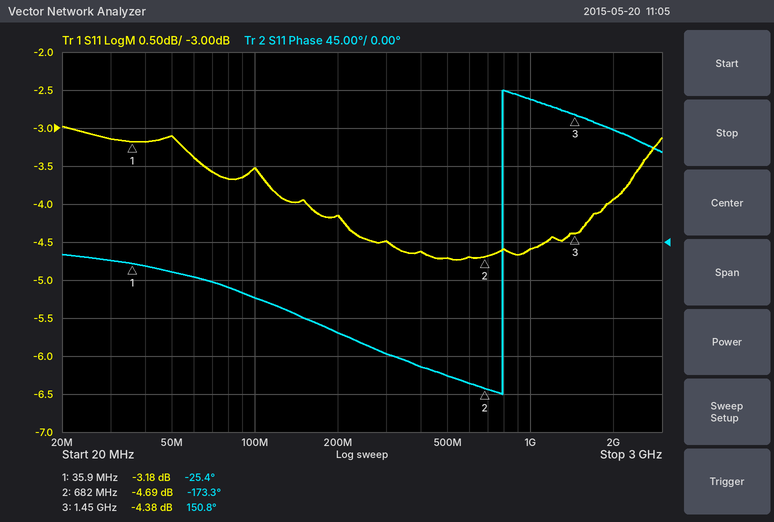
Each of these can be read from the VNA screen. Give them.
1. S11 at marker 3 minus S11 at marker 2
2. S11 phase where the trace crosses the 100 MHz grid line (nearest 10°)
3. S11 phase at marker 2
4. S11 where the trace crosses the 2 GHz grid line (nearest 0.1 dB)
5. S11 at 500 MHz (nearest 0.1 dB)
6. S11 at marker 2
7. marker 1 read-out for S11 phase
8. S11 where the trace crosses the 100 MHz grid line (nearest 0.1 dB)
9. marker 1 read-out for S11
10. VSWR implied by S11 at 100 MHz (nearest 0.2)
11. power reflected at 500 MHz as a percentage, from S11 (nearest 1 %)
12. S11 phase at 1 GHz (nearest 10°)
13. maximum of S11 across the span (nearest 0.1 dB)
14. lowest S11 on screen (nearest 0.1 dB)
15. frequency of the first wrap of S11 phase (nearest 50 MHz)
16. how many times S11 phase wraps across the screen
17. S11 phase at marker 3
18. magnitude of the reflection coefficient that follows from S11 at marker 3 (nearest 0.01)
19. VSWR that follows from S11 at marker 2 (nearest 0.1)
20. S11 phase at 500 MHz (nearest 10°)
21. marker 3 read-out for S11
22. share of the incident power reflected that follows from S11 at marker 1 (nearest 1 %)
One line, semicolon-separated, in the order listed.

0.31 dB; -70°; -173.3°; -3.9 dB; -4.7 dB; -4.69 dB; -25.4°; -3.5 dB; -3.18 dB; 5.0; 34 %; 170°; -3.0 dB; -4.7 dB; 800 MHz; 1; 150.8°; 0.60; 3.8; -160°; -4.38 dB; 48 %
